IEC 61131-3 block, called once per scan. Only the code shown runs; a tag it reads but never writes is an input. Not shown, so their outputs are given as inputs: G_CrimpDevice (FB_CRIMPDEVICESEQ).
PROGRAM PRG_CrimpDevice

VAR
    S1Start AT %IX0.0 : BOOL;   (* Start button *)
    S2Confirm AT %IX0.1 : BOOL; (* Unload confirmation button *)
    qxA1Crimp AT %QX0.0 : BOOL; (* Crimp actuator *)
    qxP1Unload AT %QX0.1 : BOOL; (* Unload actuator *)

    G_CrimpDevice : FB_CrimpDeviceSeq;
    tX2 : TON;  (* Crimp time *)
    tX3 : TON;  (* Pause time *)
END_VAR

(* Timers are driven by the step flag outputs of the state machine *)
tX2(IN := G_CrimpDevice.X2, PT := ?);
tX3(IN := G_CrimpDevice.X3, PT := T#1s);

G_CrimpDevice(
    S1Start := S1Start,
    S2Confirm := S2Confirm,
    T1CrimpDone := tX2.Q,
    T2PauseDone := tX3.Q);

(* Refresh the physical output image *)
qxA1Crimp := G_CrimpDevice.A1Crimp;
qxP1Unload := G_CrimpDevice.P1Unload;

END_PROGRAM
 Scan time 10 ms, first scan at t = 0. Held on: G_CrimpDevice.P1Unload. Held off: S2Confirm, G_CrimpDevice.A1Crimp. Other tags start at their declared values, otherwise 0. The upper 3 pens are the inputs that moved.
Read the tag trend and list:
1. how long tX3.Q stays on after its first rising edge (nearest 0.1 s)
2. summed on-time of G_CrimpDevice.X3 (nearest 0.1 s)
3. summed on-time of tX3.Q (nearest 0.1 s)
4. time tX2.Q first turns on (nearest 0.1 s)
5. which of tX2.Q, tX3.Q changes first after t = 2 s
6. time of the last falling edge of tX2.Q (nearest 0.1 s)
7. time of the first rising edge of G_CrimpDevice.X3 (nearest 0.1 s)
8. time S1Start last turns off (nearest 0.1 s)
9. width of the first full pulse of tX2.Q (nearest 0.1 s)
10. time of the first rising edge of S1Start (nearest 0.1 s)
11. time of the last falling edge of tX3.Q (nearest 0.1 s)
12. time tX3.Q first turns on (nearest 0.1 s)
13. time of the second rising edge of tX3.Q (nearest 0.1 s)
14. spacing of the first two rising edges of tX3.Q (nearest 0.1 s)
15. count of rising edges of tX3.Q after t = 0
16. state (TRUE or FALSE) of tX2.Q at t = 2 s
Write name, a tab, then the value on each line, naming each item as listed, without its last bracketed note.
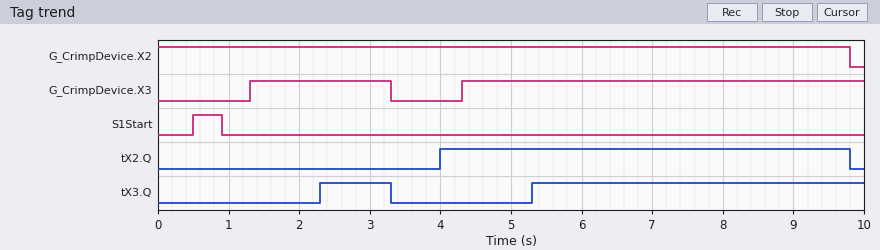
how long tX3.Q stays on after its first rising edge	1.0 s
summed on-time of G_CrimpDevice.X3	7.7 s
summed on-time of tX3.Q	5.7 s
time tX2.Q first turns on	4.0 s
which of tX2.Q, tX3.Q changes first after t = 2 s	tX3.Q
time of the last falling edge of tX2.Q	9.8 s
time of the first rising edge of G_CrimpDevice.X3	1.3 s
time S1Start last turns off	0.9 s
width of the first full pulse of tX2.Q	5.8 s
time of the first rising edge of S1Start	0.5 s
time of the last falling edge of tX3.Q	3.3 s
time tX3.Q first turns on	2.3 s
time of the second rising edge of tX3.Q	5.3 s
spacing of the first two rising edges of tX3.Q	3.0 s
count of rising edges of tX3.Q after t = 0	2
state (TRUE or FALSE) of tX2.Q at t = 2 s	FALSE
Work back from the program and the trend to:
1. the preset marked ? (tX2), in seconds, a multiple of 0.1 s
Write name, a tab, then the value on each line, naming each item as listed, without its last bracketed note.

the preset marked ? (tX2), in seconds, a multiple of 0.1 s	4.0 s
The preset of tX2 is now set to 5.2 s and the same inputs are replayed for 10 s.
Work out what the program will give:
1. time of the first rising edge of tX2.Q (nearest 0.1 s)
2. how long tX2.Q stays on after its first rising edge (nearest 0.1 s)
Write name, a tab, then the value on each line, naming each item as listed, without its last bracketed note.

time of the first rising edge of tX2.Q	5.2 s
how long tX2.Q stays on after its first rising edge	4.6 s
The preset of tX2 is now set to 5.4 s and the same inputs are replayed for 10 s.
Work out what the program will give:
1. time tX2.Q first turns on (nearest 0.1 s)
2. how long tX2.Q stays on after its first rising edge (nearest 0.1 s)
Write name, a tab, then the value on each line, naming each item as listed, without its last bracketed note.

time tX2.Q first turns on	5.4 s
how long tX2.Q stays on after its first rising edge	4.4 s
